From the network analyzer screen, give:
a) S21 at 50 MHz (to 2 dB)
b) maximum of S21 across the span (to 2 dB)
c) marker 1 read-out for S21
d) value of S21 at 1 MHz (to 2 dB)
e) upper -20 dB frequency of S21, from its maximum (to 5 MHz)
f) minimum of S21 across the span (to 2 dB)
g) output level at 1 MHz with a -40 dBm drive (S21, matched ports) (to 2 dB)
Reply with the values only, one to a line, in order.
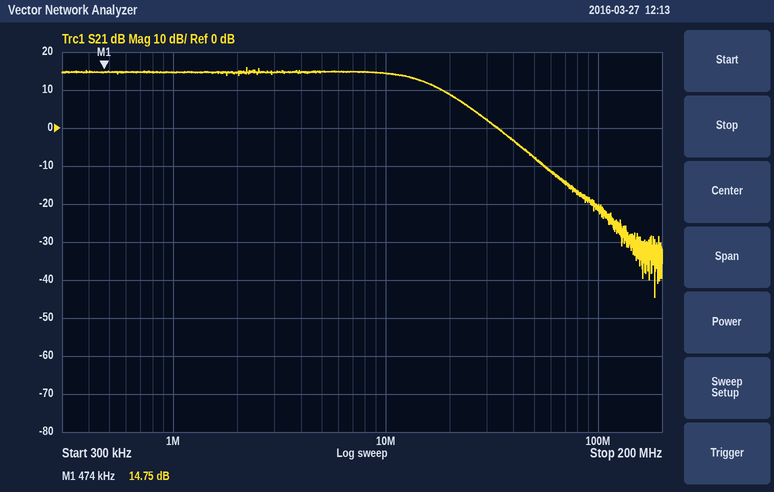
-8 dB
16 dB
14.75 dB
14 dB
40 MHz
-44 dB
-26 dBm
